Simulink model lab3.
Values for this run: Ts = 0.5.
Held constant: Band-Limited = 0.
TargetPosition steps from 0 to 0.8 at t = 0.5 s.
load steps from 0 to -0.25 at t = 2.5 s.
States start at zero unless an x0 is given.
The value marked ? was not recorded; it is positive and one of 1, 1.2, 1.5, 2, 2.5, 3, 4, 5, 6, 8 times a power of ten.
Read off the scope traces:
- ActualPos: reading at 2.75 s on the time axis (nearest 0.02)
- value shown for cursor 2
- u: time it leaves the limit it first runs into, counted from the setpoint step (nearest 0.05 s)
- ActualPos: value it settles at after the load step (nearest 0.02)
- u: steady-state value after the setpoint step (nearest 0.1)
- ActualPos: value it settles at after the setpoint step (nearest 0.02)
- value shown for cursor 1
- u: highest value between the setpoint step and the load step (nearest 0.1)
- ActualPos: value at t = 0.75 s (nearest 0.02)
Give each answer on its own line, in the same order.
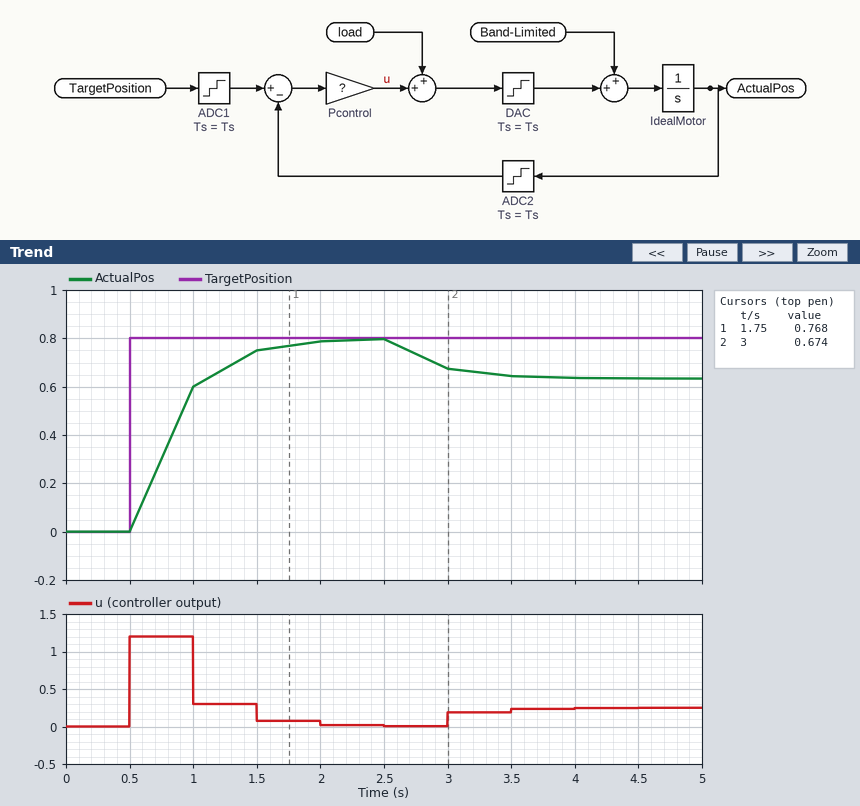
0.74
0.674
0.50 s
0.64
0.0
0.80
0.768
1.2
0.30
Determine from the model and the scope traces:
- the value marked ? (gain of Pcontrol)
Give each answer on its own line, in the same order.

1.5
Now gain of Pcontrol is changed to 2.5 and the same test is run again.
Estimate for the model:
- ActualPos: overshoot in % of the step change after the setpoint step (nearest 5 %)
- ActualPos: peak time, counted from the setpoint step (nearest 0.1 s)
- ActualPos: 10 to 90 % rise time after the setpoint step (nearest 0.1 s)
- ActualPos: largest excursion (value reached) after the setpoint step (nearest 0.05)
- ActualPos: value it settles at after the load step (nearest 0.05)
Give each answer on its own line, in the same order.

25 %
0.5 s
0.3 s
1.00
0.70
